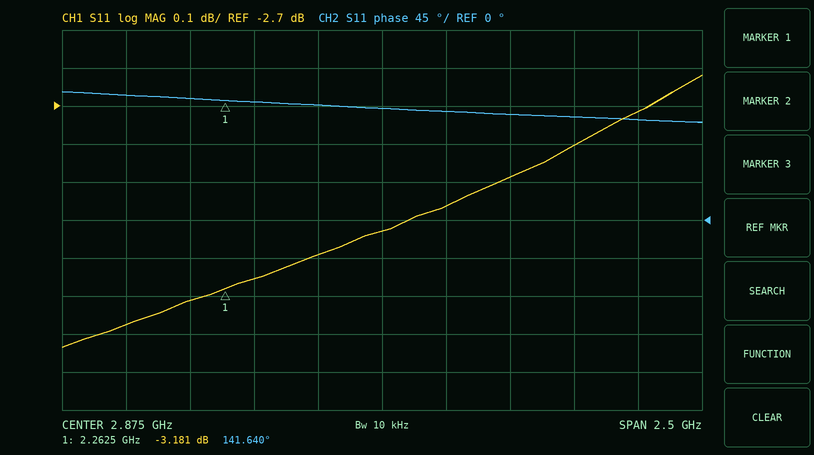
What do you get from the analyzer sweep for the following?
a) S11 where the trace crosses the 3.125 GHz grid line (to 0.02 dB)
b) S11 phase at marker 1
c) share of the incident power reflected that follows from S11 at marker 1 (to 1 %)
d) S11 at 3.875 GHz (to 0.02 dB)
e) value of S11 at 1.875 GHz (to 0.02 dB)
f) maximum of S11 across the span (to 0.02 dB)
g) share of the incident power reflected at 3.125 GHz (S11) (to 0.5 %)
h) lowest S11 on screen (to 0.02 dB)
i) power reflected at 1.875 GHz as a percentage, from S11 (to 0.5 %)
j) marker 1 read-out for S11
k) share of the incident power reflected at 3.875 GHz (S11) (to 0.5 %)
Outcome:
-2.96 dB
141.640°
48 %
-2.72 dB
-3.28 dB
-2.62 dB
50.5 %
-3.34 dB
47.0 %
-3.181 dB
53.5 %
